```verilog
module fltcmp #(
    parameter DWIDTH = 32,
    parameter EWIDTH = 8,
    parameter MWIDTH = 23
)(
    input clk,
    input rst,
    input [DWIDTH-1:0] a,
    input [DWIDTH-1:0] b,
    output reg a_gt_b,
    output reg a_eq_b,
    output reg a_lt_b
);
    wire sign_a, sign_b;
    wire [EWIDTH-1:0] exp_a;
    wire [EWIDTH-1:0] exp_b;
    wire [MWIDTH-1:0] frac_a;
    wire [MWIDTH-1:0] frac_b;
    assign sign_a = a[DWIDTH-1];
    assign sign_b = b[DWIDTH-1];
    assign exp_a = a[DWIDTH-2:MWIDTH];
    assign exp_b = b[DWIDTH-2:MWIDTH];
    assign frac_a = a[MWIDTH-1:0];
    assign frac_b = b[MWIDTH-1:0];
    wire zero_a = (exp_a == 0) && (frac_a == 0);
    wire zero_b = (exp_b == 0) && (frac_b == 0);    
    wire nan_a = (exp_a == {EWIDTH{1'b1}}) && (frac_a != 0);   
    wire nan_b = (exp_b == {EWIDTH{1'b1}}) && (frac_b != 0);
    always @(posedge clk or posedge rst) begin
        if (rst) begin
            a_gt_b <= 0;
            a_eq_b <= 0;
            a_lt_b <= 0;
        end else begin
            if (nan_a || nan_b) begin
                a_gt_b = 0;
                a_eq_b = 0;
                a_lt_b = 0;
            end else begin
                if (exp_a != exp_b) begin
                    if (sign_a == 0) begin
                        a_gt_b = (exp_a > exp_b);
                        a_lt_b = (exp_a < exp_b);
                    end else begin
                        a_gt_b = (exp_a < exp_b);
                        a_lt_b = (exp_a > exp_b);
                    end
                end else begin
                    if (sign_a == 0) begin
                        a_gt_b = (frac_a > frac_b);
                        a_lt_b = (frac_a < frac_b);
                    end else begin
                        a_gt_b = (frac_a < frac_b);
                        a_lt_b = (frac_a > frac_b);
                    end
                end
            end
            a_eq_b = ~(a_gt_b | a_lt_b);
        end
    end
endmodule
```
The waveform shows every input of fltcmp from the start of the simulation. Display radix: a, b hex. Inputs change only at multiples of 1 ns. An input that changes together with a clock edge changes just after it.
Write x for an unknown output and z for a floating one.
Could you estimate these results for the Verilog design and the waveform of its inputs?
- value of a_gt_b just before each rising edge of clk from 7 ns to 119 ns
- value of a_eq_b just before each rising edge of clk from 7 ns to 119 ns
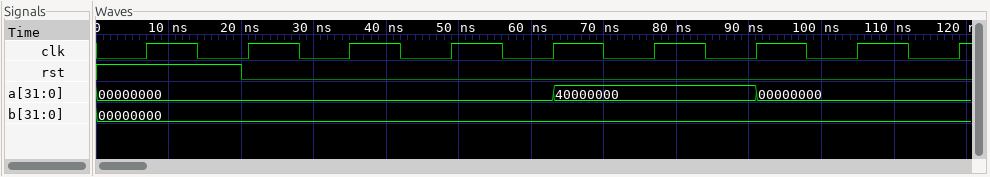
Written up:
0 0 0 0 0 0 1 1 0
0 0 1 1 1 1 0 0 1
